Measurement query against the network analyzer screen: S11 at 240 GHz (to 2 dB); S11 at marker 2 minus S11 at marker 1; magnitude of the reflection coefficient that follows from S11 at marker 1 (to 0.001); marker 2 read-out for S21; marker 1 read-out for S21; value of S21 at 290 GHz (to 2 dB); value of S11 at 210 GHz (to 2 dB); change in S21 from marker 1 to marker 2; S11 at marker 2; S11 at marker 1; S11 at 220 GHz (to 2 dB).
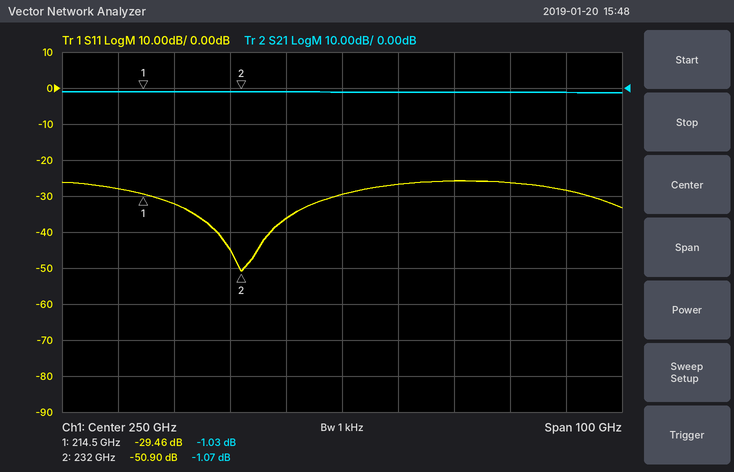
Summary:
-36 dB
-21.44 dB
0.034
-1.07 dB
-1.03 dB
-2 dB
-28 dB
-0.04 dB
-50.90 dB
-29.46 dB
-32 dB
